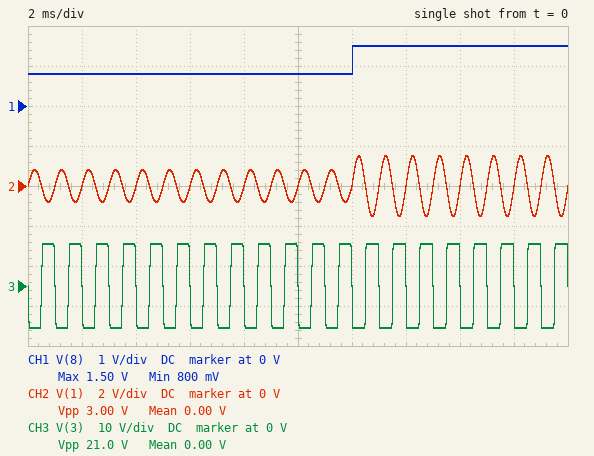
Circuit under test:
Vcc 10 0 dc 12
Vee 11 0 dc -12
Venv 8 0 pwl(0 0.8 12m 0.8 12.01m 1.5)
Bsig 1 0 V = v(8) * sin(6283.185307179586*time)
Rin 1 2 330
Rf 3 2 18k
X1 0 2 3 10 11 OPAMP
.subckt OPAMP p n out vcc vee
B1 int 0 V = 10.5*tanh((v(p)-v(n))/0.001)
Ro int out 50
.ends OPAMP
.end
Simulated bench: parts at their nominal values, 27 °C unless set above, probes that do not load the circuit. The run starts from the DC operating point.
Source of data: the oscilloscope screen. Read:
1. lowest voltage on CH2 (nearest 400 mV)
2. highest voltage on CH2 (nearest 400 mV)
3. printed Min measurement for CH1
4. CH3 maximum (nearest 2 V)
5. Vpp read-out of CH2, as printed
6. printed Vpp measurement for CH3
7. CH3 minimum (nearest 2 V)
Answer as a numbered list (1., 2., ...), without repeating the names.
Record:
1. -1.6 V
2. 1.6 V
3. 800 mV
4. 10 V
5. 3.00 V
6. 21.0 V
7. -10 V
